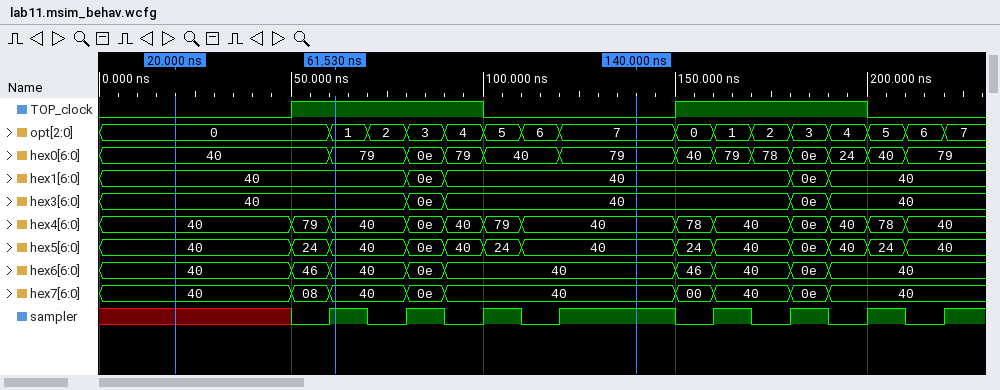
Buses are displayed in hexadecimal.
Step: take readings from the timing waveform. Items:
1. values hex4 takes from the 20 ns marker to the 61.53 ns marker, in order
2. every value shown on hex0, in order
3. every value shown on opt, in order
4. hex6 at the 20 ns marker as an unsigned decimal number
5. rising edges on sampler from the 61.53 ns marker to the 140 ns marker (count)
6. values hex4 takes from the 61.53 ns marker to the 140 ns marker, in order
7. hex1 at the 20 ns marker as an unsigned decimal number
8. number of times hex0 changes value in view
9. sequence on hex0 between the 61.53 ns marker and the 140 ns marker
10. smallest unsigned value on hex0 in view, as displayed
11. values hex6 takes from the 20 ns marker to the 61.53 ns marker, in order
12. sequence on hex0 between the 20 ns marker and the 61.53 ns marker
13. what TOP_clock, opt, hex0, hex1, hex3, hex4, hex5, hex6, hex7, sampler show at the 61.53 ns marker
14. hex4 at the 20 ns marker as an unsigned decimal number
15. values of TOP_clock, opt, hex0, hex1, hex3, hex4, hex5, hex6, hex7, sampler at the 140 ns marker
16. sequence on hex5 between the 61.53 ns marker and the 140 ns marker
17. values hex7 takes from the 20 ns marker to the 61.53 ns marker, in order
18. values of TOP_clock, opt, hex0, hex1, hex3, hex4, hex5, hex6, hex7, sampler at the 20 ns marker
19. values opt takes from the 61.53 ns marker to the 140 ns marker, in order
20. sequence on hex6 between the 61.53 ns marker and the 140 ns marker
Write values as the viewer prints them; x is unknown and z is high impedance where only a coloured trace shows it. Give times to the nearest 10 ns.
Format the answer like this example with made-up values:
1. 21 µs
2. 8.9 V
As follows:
1. 40, 79, 40
2. 40, 79, 0e, 79, 40, 79, 40, 79, 78, 0e, 24, 40, 79
3. 0, 1, 2, 3, 4, 5, 6, 7, 0, 1, 2, 3, 4, 5, 6, 7
4. 64
5. 3
6. 40, 0e, 40, 79, 40
7. 64
8. 12
9. 79, 0e, 79, 40, 79
10. 0e
11. 40, 46, 40
12. 40, 79
13. TOP_clock=1, opt=1, hex0=79, hex1=40, hex3=40, hex4=40, hex5=40, hex6=40, hex7=40, sampler=1
14. 64
15. TOP_clock=0, opt=7, hex0=79, hex1=40, hex3=40, hex4=40, hex5=40, hex6=40, hex7=40, sampler=1
16. 40, 0e, 40, 24, 40
17. 40, 08, 40
18. TOP_clock=0, opt=0, hex0=40, hex1=40, hex3=40, hex4=40, hex5=40, hex6=40, hex7=40, sampler=x
19. 1, 2, 3, 4, 5, 6, 7
20. 40, 0e, 40
